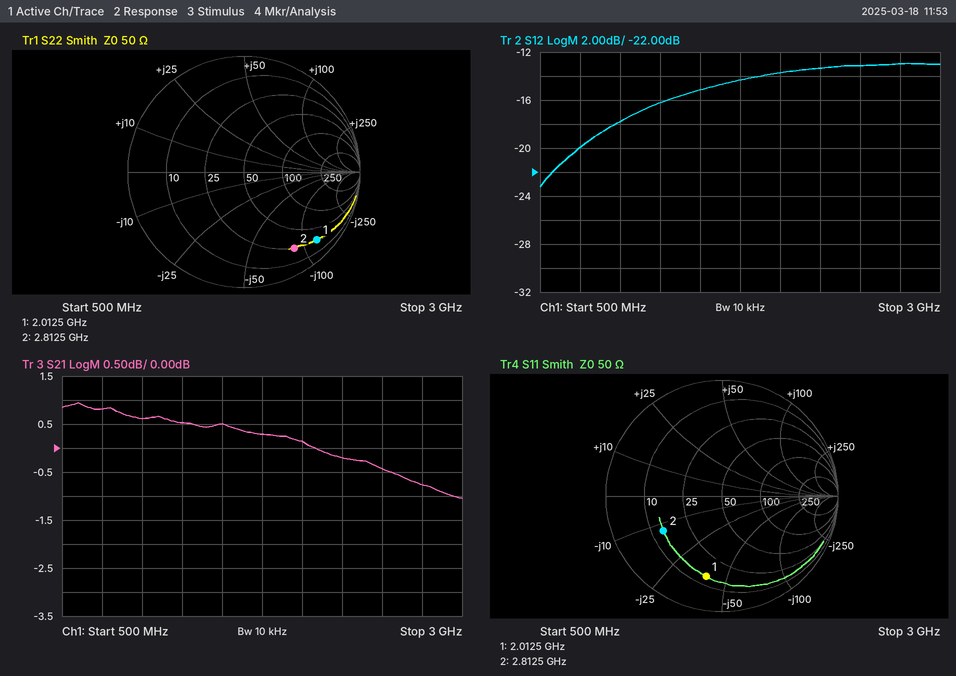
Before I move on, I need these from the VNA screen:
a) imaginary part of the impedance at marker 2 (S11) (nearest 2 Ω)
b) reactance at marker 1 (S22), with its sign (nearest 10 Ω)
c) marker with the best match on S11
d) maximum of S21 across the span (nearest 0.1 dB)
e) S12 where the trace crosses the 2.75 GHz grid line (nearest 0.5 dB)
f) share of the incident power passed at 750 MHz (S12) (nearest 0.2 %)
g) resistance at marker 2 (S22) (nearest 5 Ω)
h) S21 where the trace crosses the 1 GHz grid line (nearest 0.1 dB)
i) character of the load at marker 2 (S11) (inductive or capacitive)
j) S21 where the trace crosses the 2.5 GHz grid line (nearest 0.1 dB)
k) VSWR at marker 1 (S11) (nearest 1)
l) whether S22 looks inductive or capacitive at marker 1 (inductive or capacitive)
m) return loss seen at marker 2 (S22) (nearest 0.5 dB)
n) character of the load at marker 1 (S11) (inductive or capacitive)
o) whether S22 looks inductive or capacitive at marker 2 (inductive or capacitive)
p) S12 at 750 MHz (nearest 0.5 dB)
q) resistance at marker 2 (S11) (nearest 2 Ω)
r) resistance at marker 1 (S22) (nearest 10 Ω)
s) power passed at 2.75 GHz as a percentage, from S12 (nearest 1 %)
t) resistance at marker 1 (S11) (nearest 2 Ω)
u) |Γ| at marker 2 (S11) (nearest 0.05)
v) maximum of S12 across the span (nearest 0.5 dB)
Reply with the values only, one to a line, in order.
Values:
-12 Ω
-120 Ω
marker 2
0.9 dB
-13.0 dB
1.0 %
25 Ω
0.6 dB
capacitive
-0.4 dB
6
capacitive
2.0 dB
capacitive
capacitive
-20.0 dB
14 Ω
30 Ω
5 %
14 Ω
0.60
-13.0 dB
